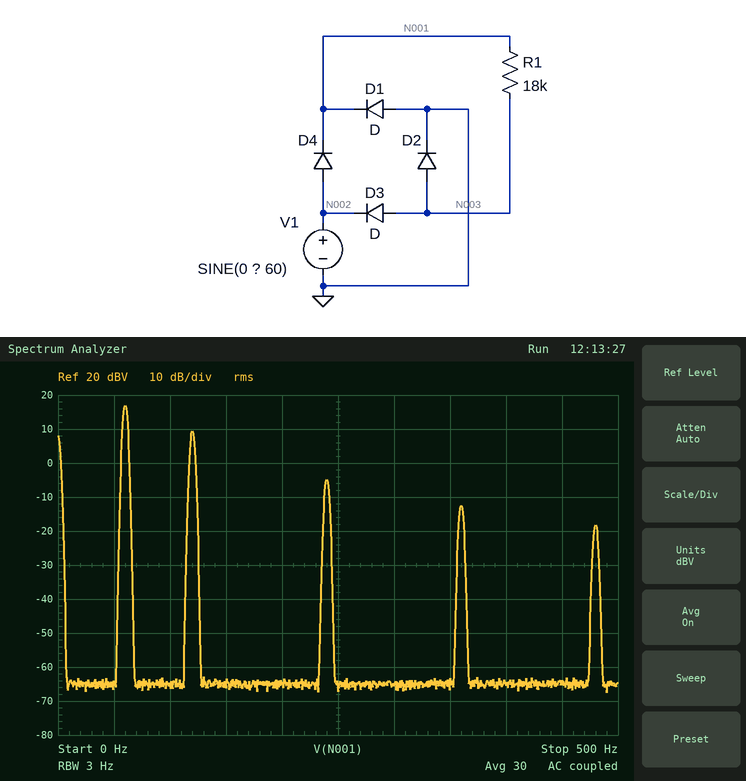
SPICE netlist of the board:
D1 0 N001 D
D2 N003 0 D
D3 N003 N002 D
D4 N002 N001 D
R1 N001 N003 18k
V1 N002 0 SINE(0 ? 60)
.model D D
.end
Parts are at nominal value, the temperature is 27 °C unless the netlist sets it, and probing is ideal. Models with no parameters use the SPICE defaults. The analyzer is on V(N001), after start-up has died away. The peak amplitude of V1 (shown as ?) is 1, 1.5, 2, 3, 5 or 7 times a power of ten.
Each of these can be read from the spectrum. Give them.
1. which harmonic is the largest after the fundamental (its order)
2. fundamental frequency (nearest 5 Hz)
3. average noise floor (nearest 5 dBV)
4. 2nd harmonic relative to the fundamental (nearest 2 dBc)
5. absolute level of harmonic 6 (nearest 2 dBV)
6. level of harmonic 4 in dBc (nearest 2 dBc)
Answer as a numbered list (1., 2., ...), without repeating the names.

1. 2
2. 60 Hz
3. -65 dBV
4. -8 dBc
5. -12 dBV
6. -22 dBc
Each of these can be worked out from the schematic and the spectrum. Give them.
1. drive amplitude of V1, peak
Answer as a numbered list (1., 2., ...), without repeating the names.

1. 20 V
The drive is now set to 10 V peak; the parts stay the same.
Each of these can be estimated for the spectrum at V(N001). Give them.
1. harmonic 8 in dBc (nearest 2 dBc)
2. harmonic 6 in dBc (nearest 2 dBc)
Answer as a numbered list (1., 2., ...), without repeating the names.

1. -38 dBc
2. -32 dBc
